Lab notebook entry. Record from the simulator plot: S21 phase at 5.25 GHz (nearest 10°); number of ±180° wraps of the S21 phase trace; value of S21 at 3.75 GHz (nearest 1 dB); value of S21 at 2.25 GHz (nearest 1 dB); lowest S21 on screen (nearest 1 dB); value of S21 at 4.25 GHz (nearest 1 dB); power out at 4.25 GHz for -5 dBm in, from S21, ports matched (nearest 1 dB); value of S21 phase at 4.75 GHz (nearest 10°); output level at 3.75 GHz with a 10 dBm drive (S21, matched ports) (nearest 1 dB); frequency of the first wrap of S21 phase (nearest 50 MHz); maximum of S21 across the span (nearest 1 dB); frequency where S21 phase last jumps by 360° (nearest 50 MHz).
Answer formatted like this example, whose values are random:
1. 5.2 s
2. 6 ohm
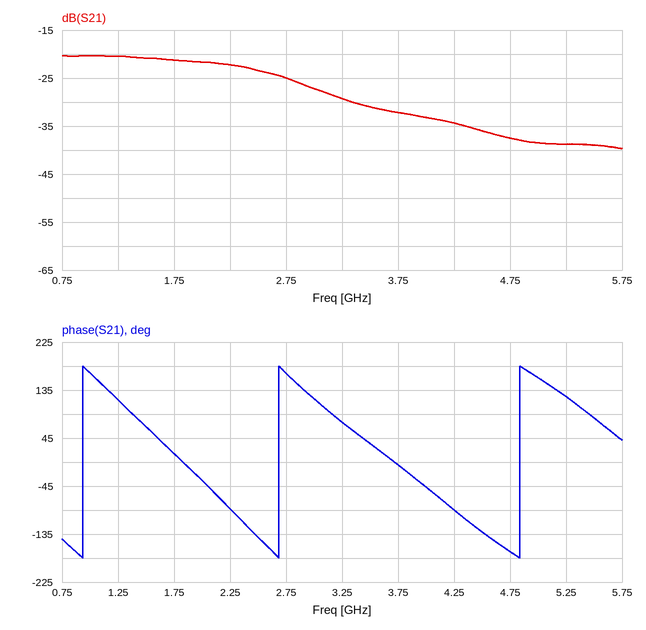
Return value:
1. 120°
2. 3
3. -32 dB
4. -22 dB
5. -40 dB
6. -34 dB
7. -39 dBm
8. -170°
9. -22 dBm
10. 950 MHz
11. -20 dB
12. 4.85 GHz
